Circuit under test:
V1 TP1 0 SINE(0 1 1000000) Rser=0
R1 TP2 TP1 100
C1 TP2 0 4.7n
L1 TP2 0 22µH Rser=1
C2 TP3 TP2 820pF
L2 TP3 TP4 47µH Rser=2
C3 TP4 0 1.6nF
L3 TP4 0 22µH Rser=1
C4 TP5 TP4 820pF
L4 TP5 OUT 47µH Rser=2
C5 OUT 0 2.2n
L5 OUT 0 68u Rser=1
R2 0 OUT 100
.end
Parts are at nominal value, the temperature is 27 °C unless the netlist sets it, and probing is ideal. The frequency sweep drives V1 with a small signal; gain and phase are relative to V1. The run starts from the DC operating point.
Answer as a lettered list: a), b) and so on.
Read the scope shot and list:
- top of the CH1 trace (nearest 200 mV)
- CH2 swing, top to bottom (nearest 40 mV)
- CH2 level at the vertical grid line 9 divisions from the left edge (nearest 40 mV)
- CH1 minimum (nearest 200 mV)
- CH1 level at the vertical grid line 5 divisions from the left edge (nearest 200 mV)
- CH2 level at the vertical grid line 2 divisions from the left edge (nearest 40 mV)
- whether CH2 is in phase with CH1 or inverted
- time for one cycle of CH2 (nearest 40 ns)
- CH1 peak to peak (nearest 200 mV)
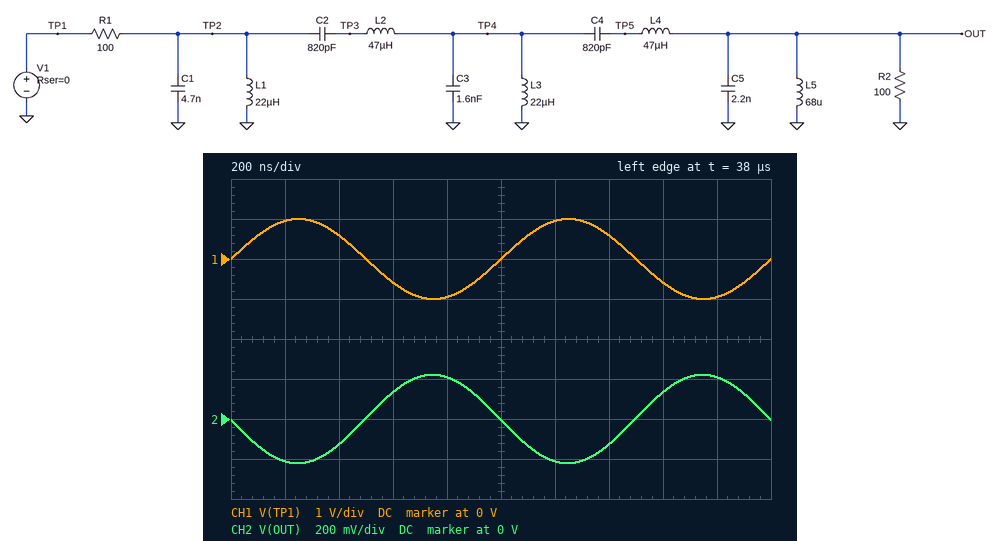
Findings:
a) 1.0 V
b) 440 mV
c) 200 mV
d) -1.0 V
e) 0 V
f) -120 mV
g) inverted
h) 1.00 µs
i) 2.0 V
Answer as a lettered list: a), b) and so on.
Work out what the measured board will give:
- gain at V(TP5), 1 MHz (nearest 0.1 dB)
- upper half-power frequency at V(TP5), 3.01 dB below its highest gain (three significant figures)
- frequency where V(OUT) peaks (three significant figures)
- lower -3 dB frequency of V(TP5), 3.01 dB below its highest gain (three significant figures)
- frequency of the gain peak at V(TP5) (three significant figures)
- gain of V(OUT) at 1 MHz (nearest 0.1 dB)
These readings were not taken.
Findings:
a) -1.5 dB
b) 1.40 MHz
c) 549 kHz
d) 1.35 MHz
e) 1.38 MHz
f) -13.1 dB
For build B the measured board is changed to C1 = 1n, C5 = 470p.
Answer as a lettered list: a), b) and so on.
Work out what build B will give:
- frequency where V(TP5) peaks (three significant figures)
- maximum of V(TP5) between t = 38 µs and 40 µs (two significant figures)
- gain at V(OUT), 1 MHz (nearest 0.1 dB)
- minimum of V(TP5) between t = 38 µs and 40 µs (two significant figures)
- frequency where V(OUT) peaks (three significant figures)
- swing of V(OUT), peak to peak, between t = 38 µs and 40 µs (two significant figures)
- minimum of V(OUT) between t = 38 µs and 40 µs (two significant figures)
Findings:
a) 1.33 MHz
b) 1.2 V
c) -8.1 dB
d) -1.2 V
e) 1.31 MHz
f) 790 mV
g) -390 mV
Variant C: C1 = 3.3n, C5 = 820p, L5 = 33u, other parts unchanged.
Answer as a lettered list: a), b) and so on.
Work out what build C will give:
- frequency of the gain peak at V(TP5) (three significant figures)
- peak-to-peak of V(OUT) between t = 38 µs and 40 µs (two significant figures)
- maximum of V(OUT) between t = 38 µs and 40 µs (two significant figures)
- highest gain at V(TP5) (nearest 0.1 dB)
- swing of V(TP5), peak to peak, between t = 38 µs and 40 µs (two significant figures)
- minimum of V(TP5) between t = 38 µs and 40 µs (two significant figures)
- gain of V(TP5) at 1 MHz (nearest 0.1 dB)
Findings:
a) 1.36 MHz
b) 640 mV
c) 320 mV
d) 3.3 dB
e) 2.0 V
f) -990 mV
g) -0.1 dB
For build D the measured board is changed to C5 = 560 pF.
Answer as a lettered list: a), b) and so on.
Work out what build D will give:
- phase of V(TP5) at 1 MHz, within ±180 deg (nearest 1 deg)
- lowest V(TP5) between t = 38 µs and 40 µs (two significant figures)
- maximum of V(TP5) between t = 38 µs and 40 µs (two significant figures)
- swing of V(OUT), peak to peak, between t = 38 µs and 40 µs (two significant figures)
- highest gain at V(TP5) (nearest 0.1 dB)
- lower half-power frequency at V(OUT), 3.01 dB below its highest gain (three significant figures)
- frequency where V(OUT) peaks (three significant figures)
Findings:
a) -51 deg
b) -710 mV
c) 710 mV
d) 470 mV
e) 0.6 dB
f) 483 kHz
g) 536 kHz
